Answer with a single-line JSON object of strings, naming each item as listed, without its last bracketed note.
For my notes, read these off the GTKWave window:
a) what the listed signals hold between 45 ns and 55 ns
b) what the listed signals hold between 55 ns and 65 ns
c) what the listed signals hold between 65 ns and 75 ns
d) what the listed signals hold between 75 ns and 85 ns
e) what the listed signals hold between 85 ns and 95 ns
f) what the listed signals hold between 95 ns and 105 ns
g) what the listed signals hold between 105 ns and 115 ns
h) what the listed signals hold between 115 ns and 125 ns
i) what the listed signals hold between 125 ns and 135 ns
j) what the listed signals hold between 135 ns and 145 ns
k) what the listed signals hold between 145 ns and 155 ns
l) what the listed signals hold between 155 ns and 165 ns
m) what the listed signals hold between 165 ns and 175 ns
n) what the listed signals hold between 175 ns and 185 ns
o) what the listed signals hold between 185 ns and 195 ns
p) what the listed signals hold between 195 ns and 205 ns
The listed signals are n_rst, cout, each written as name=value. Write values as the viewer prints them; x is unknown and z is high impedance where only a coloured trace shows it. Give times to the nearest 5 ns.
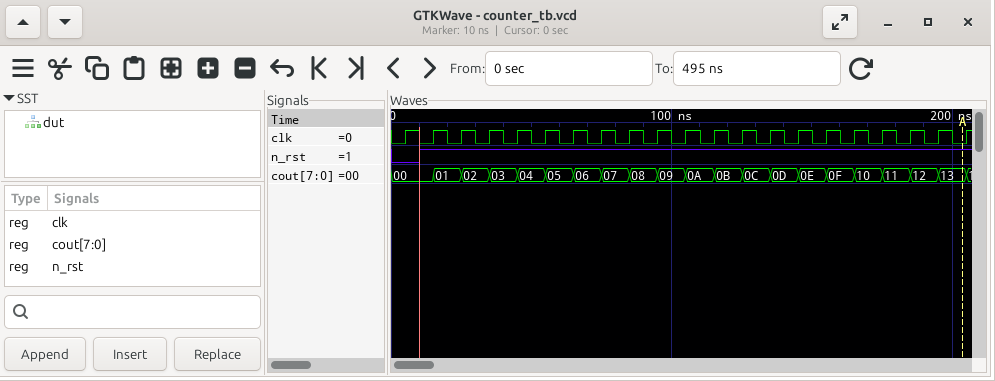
{"what the listed signals hold between 45 ns and 55 ns": "n_rst=1, cout=04", "what the listed signals hold between 55 ns and 65 ns": "n_rst=1, cout=05", "what the listed signals hold between 65 ns and 75 ns": "n_rst=1, cout=06", "what the listed signals hold between 75 ns and 85 ns": "n_rst=1, cout=07", "what the listed signals hold between 85 ns and 95 ns": "n_rst=1, cout=08", "what the listed signals hold between 95 ns and 105 ns": "n_rst=1, cout=09", "what the listed signals hold between 105 ns and 115 ns": "n_rst=1, cout=0A", "what the listed signals hold between 115 ns and 125 ns": "n_rst=1, cout=0B", "what the listed signals hold between 125 ns and 135 ns": "n_rst=1, cout=0C", "what the listed signals hold between 135 ns and 145 ns": "n_rst=1, cout=0D", "what the listed signals hold between 145 ns and 155 ns": "n_rst=1, cout=0E", "what the listed signals hold between 155 ns and 165 ns": "n_rst=1, cout=0F", "what the listed signals hold between 165 ns and 175 ns": "n_rst=1, cout=10", "what the listed signals hold between 175 ns and 185 ns": "n_rst=1, cout=11", "what the listed signals hold between 185 ns and 195 ns": "n_rst=1, cout=12", "what the listed signals hold between 195 ns and 205 ns": "n_rst=1, cout=13"}
